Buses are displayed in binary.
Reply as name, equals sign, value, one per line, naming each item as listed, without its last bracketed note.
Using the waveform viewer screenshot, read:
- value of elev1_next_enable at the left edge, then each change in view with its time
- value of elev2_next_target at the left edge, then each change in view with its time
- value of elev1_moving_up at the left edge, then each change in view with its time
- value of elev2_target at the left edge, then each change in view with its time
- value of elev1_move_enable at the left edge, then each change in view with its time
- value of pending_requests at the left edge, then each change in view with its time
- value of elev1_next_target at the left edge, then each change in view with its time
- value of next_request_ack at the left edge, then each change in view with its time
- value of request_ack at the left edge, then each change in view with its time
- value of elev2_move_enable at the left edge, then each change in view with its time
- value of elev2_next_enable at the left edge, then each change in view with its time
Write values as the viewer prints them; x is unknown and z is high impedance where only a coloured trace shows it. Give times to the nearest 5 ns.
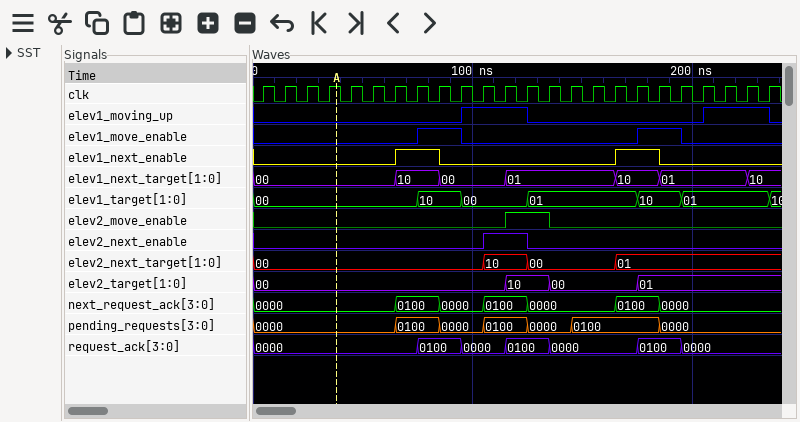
value of elev1_next_enable at the left edge, then each change in view with its time = 0, 1 at 65 ns, 0 at 85 ns, 1 at 165 ns, 0 at 185 ns
value of elev2_next_target at the left edge, then each change in view with its time = 00, 10 at 105 ns, 00 at 125 ns, 01 at 165 ns
value of elev1_moving_up at the left edge, then each change in view with its time = 0, 1 at 95 ns, 0 at 125 ns, 1 at 205 ns, 0 at 235 ns
value of elev2_target at the left edge, then each change in view with its time = 00, 10 at 115 ns, 00 at 135 ns, 01 at 175 ns
value of elev1_move_enable at the left edge, then each change in view with its time = 0, 1 at 75 ns, 0 at 95 ns, 1 at 175 ns, 0 at 195 ns
value of pending_requests at the left edge, then each change in view with its time = 0000, 0100 at 65 ns, 0000 at 85 ns, 0100 at 105 ns, 0000 at 125 ns, 0100 at 145 ns, 0000 at 185 ns
value of elev1_next_target at the left edge, then each change in view with its time = 00, 10 at 65 ns, 00 at 85 ns, 01 at 115 ns, 10 at 165 ns, 01 at 185 ns, 10 at 225 ns
value of next_request_ack at the left edge, then each change in view with its time = 0000, 0100 at 65 ns, 0000 at 85 ns, 0100 at 105 ns, 0000 at 125 ns, 0100 at 165 ns, 0000 at 185 ns
value of request_ack at the left edge, then each change in view with its time = 0000, 0100 at 75 ns, 0000 at 95 ns, 0100 at 115 ns, 0000 at 135 ns, 0100 at 175 ns, 0000 at 195 ns
value of elev2_move_enable at the left edge, then each change in view with its time = 0, 1 at 115 ns, 0 at 135 ns
value of elev2_next_enable at the left edge, then each change in view with its time = 0, 1 at 105 ns, 0 at 125 ns
